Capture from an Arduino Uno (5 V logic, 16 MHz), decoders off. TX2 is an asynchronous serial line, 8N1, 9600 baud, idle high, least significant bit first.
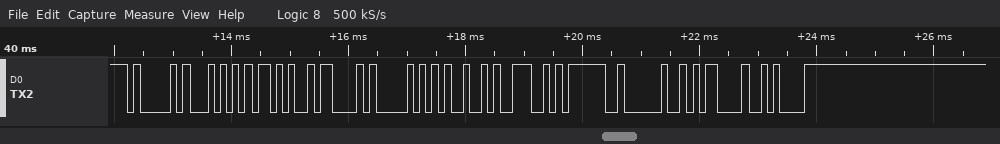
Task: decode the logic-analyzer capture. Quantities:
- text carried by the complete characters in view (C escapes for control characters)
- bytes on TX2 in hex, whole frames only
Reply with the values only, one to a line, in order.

"AT+CPIN? \r\n"
0x41 0x54 0x2B 0x43 0x50 0x49 0x4E 0x3F 0x20 0x0D 0x0A
